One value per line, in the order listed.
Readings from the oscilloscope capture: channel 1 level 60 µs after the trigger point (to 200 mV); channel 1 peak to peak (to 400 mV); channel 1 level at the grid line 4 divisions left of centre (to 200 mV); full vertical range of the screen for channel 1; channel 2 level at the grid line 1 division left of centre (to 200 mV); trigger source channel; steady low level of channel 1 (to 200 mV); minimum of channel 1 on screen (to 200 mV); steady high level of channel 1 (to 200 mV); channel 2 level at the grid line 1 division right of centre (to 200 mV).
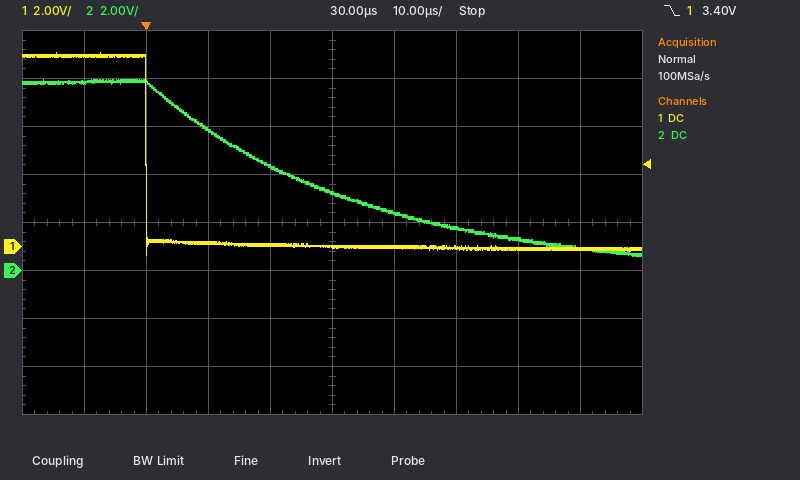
0.0 V
8.4 V
8.0 V
16 V
4.4 V
channel 1
0.0 V
-400 mV
8.0 V
2.4 V
